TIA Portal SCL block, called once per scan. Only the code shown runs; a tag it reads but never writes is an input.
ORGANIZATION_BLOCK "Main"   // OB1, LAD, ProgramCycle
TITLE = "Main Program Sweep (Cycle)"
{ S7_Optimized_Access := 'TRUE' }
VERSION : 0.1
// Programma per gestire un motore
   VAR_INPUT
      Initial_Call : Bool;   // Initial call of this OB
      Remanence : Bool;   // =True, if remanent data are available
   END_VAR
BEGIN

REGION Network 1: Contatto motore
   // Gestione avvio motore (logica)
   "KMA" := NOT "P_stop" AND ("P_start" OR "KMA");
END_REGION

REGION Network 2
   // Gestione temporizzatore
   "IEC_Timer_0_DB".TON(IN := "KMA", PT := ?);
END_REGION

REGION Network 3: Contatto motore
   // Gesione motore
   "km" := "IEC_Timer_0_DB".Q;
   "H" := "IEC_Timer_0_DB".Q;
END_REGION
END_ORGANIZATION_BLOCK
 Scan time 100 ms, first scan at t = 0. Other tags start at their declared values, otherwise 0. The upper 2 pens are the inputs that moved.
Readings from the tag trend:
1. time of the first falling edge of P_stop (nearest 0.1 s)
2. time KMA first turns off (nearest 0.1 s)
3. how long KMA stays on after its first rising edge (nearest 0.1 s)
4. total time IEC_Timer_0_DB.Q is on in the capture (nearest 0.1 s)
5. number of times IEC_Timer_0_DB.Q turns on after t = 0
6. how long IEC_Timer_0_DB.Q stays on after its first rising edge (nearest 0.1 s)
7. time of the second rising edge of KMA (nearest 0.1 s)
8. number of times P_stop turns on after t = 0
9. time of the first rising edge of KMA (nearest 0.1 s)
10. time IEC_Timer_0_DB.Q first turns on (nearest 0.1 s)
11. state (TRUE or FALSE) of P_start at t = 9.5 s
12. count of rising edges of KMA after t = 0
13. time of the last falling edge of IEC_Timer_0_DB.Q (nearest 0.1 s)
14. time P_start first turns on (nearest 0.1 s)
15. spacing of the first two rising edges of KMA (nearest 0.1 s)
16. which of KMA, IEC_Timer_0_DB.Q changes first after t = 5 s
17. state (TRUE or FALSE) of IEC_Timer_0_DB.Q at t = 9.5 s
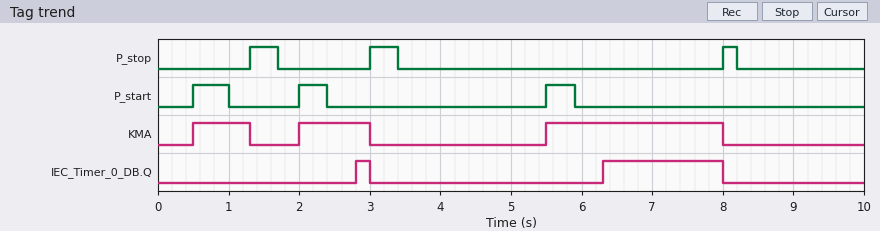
1.7 s
1.3 s
0.8 s
1.9 s
2
0.2 s
2.0 s
3
0.5 s
2.8 s
FALSE
3
8.0 s
0.5 s
1.5 s
KMA
FALSE
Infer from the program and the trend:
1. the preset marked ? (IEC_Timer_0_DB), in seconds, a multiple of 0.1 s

0.8 s
